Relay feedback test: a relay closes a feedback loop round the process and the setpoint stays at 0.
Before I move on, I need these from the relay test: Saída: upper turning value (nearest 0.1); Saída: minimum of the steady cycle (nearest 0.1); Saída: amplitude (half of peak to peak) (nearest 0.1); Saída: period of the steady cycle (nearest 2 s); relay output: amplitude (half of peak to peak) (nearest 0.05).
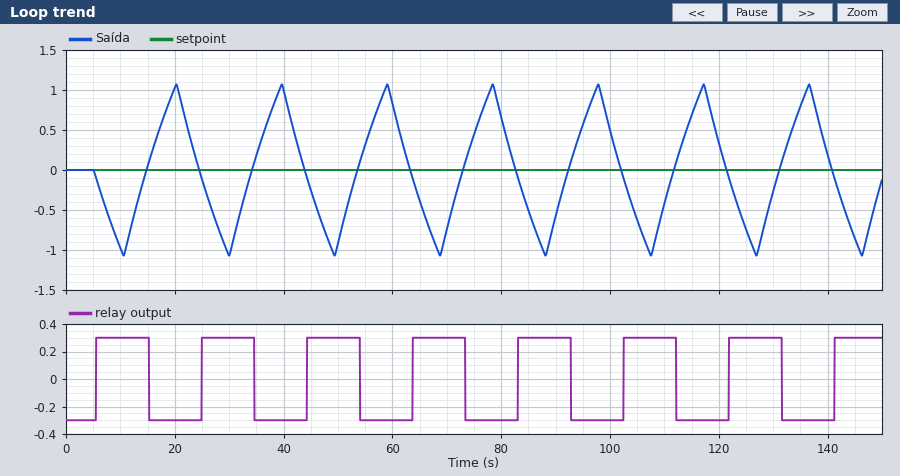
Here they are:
1.1
-1.1
1.1
20 s
0.30
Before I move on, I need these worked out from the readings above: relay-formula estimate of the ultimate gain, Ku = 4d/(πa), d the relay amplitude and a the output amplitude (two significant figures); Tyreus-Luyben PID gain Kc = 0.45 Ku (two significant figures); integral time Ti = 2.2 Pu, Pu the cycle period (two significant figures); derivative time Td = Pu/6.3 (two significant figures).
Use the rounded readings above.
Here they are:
0.35
0.16
44 s
3.2 s
